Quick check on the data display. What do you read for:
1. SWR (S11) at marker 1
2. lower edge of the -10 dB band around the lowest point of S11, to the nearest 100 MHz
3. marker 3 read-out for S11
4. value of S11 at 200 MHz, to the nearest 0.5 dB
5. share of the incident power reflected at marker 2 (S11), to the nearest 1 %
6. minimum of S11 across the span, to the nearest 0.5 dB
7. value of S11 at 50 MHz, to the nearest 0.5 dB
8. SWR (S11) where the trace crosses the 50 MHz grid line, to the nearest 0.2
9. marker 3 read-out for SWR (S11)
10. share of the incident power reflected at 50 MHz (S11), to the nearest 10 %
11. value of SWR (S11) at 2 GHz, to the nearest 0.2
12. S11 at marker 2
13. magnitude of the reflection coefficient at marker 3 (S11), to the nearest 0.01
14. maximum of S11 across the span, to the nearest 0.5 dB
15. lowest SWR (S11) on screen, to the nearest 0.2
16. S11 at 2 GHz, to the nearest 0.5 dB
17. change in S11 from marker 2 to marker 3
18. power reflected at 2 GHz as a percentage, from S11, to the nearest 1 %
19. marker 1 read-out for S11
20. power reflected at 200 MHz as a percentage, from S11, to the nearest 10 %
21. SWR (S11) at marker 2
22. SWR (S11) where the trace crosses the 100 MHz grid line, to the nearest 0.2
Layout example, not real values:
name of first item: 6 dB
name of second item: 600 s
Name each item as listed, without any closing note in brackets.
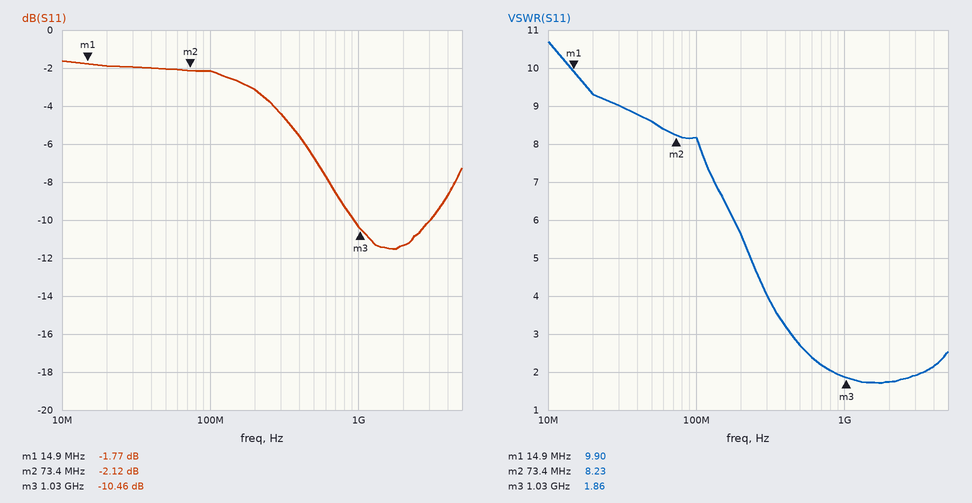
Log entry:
SWR (S11) at marker 1: 9.90
lower edge of the -10 dB band around the lowest point of S11, to the nearest 100 MHz: 900 MHz
marker 3 read-out for S11: -10.46 dB
value of S11 at 200 MHz, to the nearest 0.5 dB: -3.0 dB
share of the incident power reflected at marker 2 (S11), to the nearest 1 %: 61 %
minimum of S11 across the span, to the nearest 0.5 dB: -11.5 dB
value of S11 at 50 MHz, to the nearest 0.5 dB: -2.0 dB
SWR (S11) where the trace crosses the 50 MHz grid line, to the nearest 0.2: 8.6
marker 3 read-out for SWR: 1.86
share of the incident power reflected at 50 MHz (S11), to the nearest 10 %: 60 %
value of SWR (S11) at 2 GHz, to the nearest 0.2: 1.8
S11 at marker 2: -2.12 dB
magnitude of the reflection coefficient at marker 3 (S11), to the nearest 0.01: 0.30
maximum of S11 across the span, to the nearest 0.5 dB: -1.5 dB
lowest SWR (S11) on screen, to the nearest 0.2: 1.8
S11 at 2 GHz, to the nearest 0.5 dB: -11.5 dB
change in S11 from marker 2 to marker 3: -8.34 dB
power reflected at 2 GHz as a percentage, from S11, to the nearest 1 %: 7 %
marker 1 read-out for S11: -1.77 dB
power reflected at 200 MHz as a percentage, from S11, to the nearest 10 %: 50 %
SWR (S11) at marker 2: 8.23
SWR (S11) where the trace crosses the 100 MHz grid line, to the nearest 0.2: 8.2
